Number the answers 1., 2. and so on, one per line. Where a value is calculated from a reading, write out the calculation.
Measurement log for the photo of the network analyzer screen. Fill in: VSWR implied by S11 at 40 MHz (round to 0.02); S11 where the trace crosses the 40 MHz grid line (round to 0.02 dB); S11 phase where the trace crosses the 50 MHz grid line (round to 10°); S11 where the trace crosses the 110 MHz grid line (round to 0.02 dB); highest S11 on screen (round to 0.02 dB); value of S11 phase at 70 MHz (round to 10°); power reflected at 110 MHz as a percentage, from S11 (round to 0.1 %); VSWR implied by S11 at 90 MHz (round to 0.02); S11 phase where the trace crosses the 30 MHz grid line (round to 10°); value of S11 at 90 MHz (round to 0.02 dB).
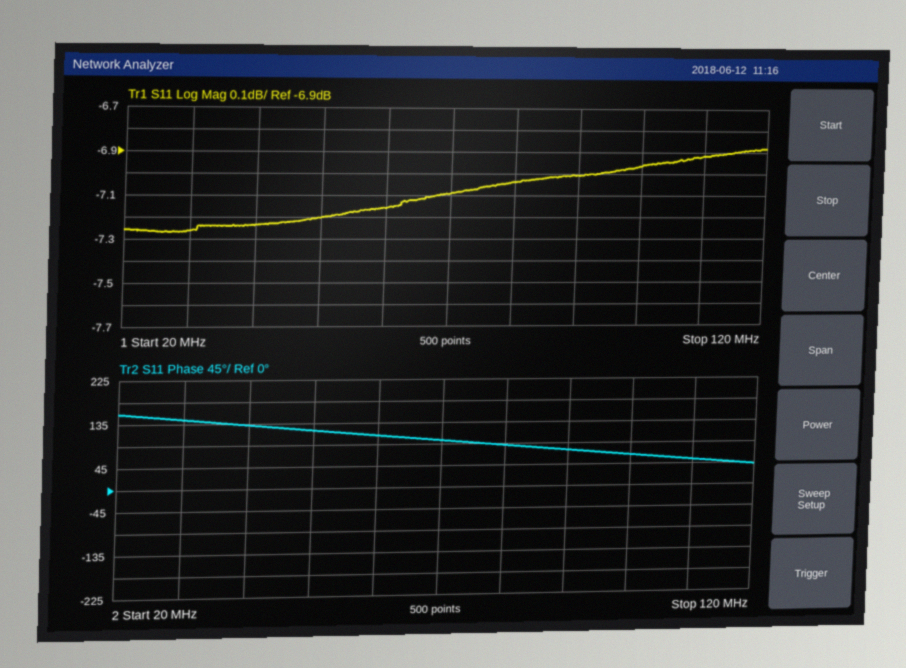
1. |Γ| = 10^(-7.24/20) = 0.4345; VSWR = (1 + 0.4345)/(1 − 0.4345) ≈ 2.54
2. -7.24 dB
3. 120°
4. -6.92 dB
5. -6.88 dB
6. 100°
7. 10^(-6.92/10) ≈ 20.3 %
8. |Γ| = 10^(-7/20) = 0.4467; VSWR = (1 + 0.4467)/(1 − 0.4467) ≈ 2.61, so 2.62 to the nearest 0.02
9. 140°
10. -7.00 dB
